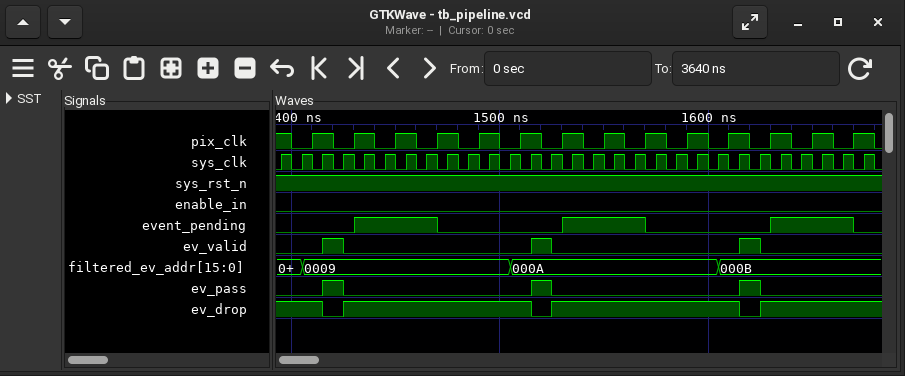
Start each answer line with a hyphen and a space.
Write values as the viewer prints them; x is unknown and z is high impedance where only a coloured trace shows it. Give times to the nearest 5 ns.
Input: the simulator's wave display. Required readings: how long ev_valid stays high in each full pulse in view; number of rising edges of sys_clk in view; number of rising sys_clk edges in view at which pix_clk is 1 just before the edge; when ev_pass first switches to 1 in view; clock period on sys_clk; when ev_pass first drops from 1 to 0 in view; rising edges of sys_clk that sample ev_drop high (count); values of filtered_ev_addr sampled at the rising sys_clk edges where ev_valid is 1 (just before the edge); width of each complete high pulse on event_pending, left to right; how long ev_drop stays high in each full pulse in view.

- 10 ns, 10 ns, 10 ns
- 29
- 15
- 1415 ns
- 10 ns
- 1425 ns
- 26
- 0009, 000A, 000B
- 40 ns, 40 ns, 40 ns
- 90 ns, 90 ns
